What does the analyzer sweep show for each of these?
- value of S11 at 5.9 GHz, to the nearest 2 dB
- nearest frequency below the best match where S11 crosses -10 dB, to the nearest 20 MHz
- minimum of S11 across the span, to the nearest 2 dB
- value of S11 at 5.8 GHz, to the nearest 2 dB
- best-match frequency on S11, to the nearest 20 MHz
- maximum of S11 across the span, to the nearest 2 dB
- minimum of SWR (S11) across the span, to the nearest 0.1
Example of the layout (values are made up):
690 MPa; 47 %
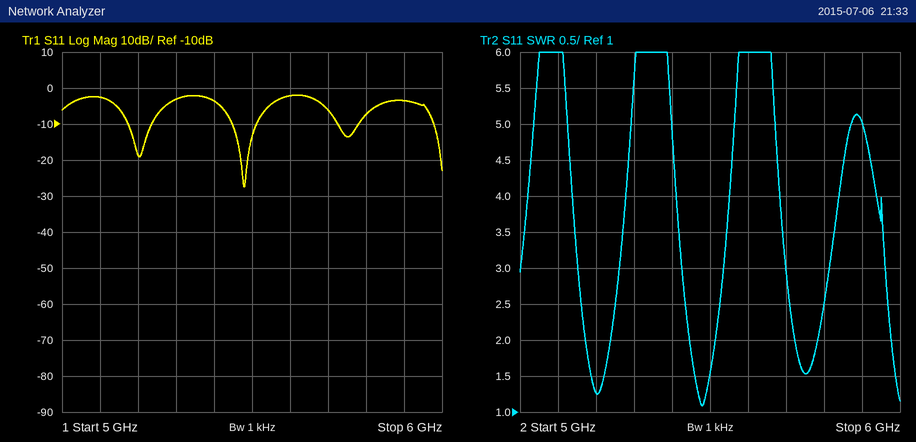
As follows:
-4 dB; 5.44 GHz; -28 dB; -8 dB; 5.48 GHz; -2 dB; 1.1
